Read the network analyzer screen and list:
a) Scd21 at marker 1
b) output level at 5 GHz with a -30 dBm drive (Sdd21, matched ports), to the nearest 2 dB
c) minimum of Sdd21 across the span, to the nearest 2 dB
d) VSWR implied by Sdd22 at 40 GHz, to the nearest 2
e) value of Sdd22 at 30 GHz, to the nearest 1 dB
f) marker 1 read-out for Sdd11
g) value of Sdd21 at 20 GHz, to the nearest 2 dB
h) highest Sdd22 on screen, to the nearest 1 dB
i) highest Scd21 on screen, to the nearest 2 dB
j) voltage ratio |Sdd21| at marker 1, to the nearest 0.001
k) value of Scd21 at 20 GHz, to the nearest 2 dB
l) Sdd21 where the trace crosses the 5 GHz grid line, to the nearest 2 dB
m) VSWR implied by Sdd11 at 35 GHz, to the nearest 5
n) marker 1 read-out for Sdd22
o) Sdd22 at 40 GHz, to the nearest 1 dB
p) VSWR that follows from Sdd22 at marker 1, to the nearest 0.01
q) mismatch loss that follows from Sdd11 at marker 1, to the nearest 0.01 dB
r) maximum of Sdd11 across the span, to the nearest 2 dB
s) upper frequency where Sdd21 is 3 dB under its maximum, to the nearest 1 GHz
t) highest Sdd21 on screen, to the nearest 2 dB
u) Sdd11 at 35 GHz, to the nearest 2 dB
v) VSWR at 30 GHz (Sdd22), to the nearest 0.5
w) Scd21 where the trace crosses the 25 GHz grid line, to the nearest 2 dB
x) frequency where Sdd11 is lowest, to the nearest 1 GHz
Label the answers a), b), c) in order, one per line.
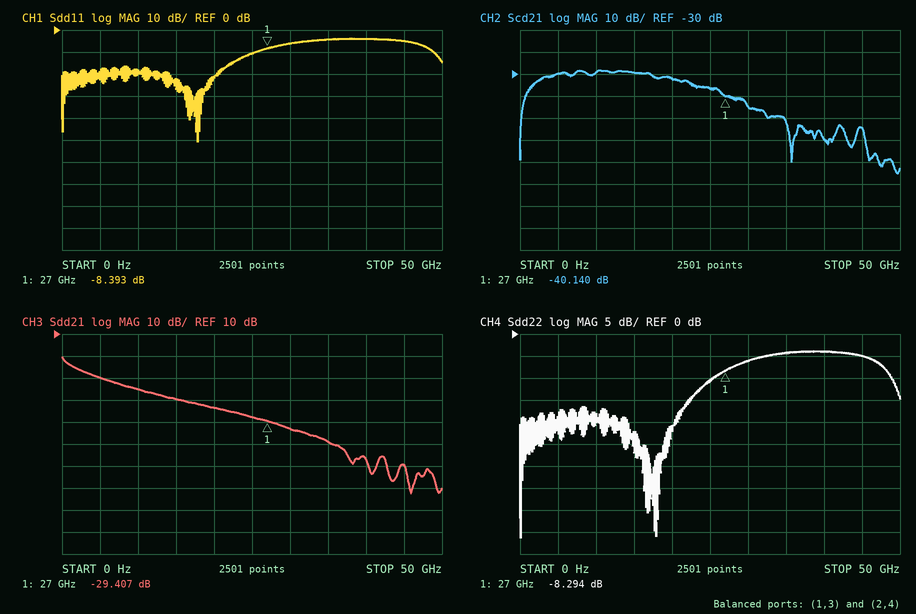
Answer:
a) -40.140 dB
b) -40 dBm
c) -62 dB
d) 4
e) -6 dB
f) -8.393 dB
g) -24 dB
h) -4 dB
i) -28 dB
j) 0.034
k) -32 dB
l) -10 dB
m) 5
n) -8.294 dB
o) -4 dB
p) 2.25
q) 0.68 dB
r) -4 dB
s) 1 GHz
t) 0 dB
u) -4 dB
v) 3.0
w) -36 dB
x) 18 GHz
